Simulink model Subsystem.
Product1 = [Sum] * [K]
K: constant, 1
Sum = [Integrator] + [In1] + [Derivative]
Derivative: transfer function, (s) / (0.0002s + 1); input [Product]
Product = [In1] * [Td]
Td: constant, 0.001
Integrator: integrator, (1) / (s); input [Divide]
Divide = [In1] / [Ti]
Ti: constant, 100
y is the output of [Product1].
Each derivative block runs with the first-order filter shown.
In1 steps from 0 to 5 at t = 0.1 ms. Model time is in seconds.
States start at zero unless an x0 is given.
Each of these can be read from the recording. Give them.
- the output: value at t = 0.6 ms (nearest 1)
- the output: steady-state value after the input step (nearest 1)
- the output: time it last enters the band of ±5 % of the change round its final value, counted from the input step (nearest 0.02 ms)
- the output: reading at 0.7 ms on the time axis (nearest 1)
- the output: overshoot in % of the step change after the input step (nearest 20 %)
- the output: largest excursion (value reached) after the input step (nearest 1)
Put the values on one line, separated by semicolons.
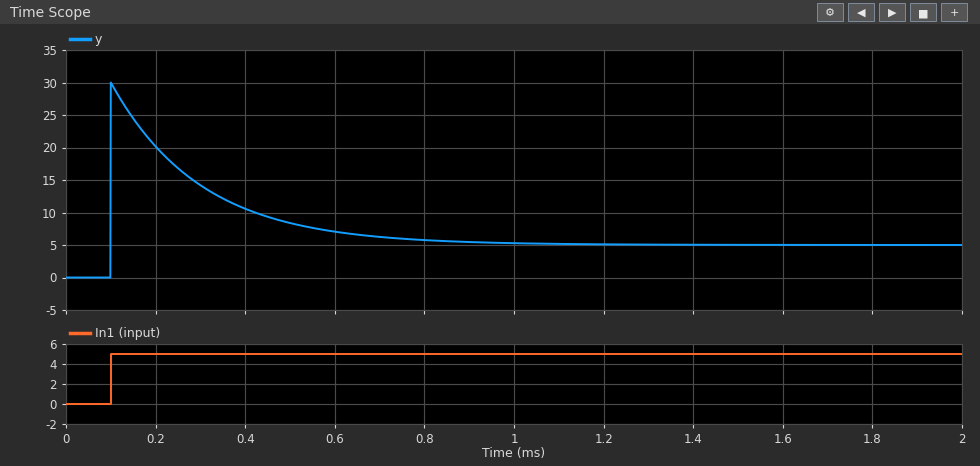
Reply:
7; 5; 0.92 ms; 6; 500 %; 30
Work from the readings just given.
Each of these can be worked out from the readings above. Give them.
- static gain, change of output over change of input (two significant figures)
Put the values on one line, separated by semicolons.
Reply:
1.0
